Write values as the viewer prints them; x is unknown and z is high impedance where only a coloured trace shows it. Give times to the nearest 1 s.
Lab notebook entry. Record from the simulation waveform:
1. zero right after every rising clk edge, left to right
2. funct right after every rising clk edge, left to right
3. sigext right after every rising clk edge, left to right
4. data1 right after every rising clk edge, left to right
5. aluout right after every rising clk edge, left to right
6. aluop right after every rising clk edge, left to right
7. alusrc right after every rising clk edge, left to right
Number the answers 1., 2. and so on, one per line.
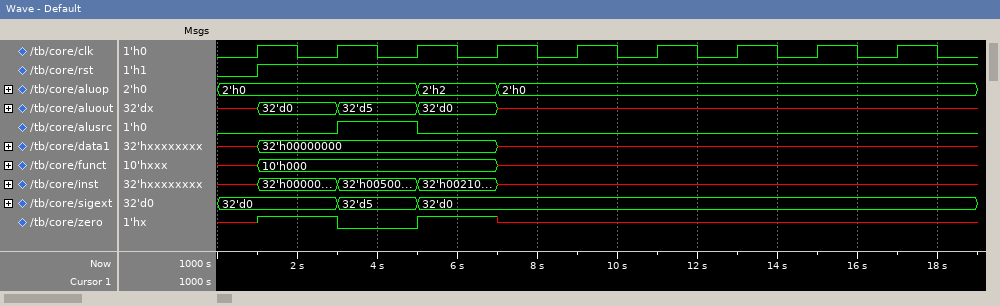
1. 1 0 1 x x x x x x
2. 10'h000, 10'h000, 10'h000, x, x, x, x, x, x
3. 32'd0, 32'd5, 32'd0, 32'd0, 32'd0, 32'd0, 32'd0, 32'd0, 32'd0
4. 32'h00000000, 32'h00000000, 32'h00000000, x, x, x, x, x, x
5. 32'd0, 32'd5, 32'd0, x, x, x, x, x, x
6. 2'h0, 2'h0, 2'h2, 2'h0, 2'h0, 2'h0, 2'h0, 2'h0, 2'h0
7. 0 1 0 0 0 0 0 0 0
